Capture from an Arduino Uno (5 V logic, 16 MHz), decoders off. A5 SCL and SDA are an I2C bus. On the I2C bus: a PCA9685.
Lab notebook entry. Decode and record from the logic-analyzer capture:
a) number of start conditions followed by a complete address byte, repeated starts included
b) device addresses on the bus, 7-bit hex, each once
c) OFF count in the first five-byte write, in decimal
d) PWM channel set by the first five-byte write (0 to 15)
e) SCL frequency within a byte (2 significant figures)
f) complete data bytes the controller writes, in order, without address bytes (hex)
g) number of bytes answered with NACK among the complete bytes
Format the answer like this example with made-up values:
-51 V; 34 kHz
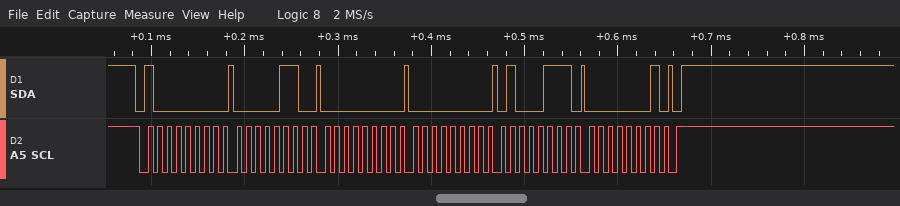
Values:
1; 0x40; 327; 0; 100 kHz; 06 00 00 47 01; 0
